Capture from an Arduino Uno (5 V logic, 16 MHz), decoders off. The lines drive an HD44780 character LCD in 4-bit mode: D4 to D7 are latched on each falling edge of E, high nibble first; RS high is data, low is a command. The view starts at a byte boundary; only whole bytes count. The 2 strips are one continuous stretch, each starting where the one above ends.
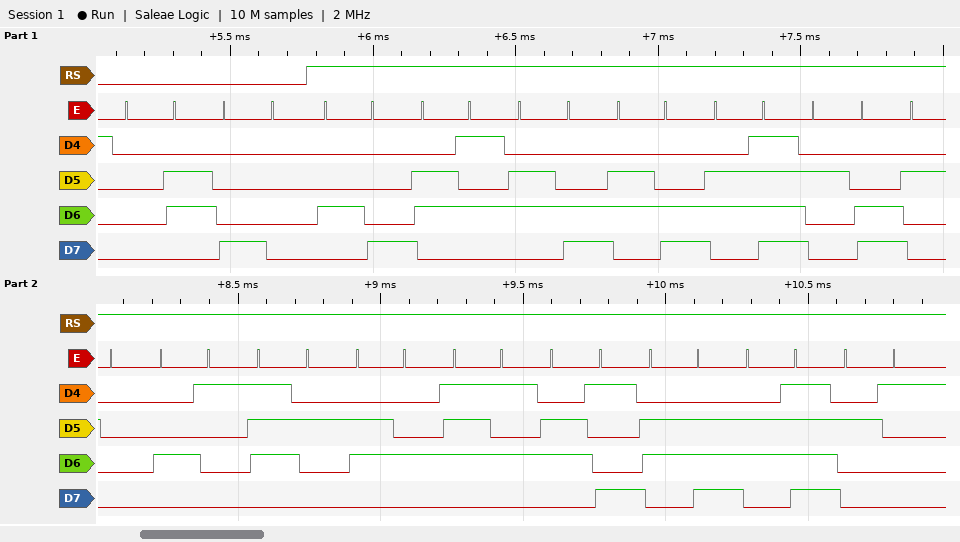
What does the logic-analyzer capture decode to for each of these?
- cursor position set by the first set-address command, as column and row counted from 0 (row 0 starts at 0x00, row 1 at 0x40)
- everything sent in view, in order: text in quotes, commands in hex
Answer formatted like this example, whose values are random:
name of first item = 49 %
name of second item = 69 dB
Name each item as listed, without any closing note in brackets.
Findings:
cursor position set by the first set-address command, as column and row counted from 0 = column 0, row 0
everything sent in view, in order: text in quotes, commands in hex = 0x06 0x80 "Hello, Arduino!"
